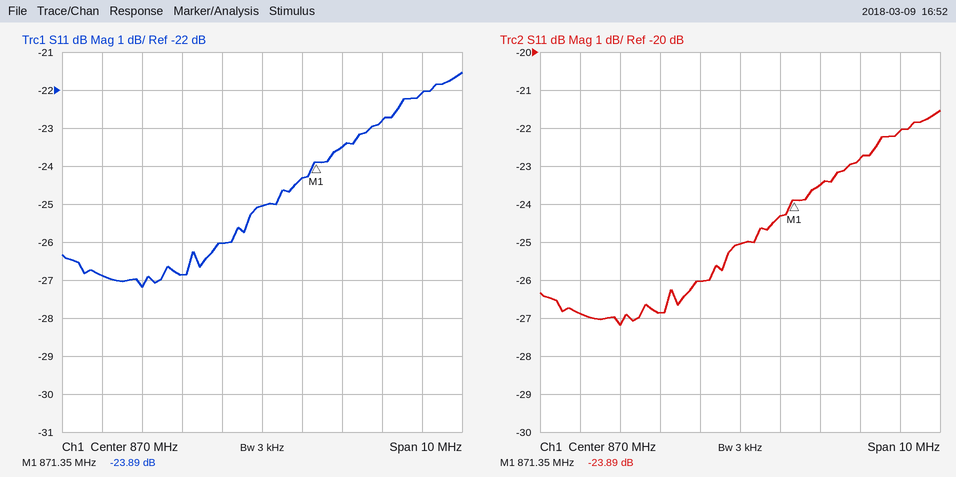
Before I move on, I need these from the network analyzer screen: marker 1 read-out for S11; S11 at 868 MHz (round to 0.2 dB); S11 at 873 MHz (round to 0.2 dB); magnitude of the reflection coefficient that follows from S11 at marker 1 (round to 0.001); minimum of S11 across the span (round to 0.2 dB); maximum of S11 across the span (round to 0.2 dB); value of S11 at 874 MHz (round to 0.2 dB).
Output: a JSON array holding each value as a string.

["-23.89 dB", "-26.8 dB", "-22.8 dB", "0.064", "-27.2 dB", "-21.6 dB", "-22.0 dB"]
